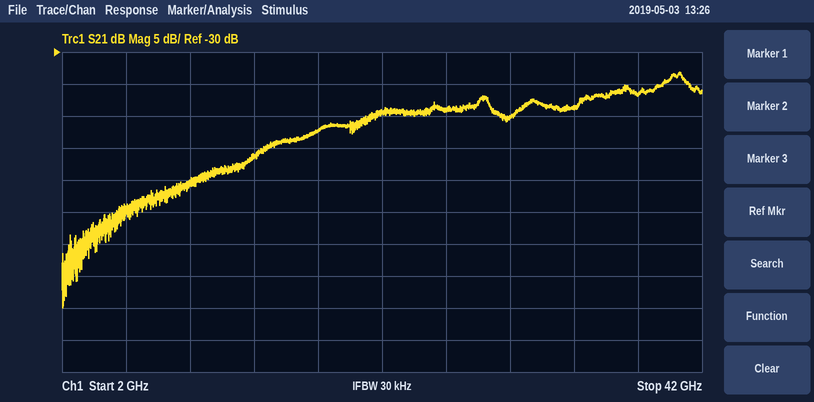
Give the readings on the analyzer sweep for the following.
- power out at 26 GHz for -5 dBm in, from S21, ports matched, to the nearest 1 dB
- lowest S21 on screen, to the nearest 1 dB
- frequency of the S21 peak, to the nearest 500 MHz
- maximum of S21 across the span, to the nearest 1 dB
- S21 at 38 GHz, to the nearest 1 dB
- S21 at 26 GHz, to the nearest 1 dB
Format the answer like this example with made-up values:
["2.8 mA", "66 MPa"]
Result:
["-44 dBm", "-70 dB", "40.5 GHz", "-33 dB", "-37 dB", "-39 dB"]
